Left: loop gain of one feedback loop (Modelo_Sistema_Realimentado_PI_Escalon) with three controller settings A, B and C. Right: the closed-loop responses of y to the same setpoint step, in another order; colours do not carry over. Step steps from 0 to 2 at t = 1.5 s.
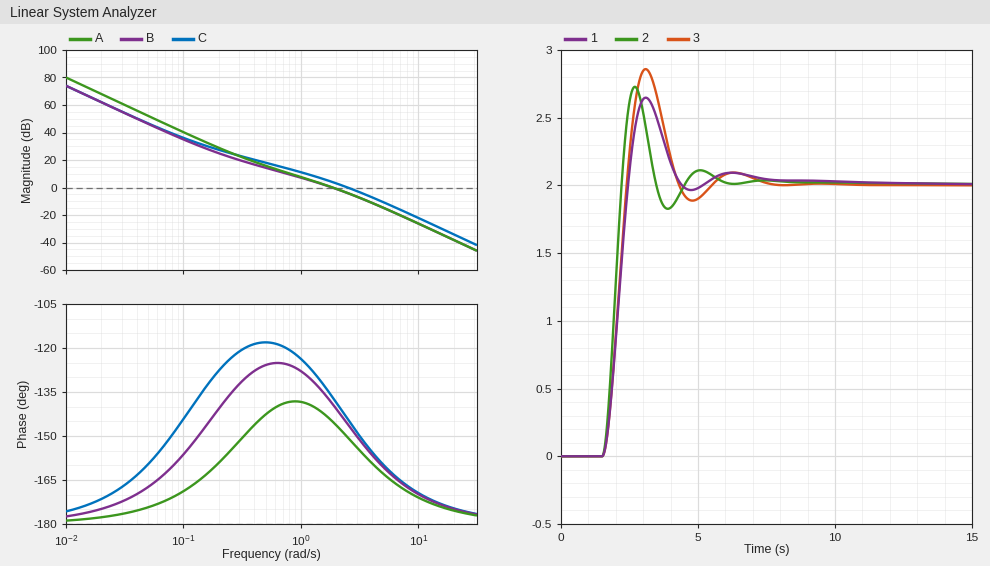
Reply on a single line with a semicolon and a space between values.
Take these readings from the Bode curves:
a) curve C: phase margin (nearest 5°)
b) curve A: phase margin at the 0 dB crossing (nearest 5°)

35°; 35°
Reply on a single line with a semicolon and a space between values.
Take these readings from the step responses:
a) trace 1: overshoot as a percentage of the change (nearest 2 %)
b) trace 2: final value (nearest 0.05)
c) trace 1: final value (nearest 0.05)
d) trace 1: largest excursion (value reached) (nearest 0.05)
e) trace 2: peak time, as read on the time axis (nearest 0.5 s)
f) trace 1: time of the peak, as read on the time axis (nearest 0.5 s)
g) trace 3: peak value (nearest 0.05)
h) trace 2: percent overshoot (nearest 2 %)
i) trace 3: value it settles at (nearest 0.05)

32 %; 2.00; 2.00; 2.65; 2.5 s; 3.0 s; 2.85; 36 %; 2.00
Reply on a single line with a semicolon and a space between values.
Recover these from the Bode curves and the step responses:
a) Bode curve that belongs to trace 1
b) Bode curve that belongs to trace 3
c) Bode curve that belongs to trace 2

B; A; C
